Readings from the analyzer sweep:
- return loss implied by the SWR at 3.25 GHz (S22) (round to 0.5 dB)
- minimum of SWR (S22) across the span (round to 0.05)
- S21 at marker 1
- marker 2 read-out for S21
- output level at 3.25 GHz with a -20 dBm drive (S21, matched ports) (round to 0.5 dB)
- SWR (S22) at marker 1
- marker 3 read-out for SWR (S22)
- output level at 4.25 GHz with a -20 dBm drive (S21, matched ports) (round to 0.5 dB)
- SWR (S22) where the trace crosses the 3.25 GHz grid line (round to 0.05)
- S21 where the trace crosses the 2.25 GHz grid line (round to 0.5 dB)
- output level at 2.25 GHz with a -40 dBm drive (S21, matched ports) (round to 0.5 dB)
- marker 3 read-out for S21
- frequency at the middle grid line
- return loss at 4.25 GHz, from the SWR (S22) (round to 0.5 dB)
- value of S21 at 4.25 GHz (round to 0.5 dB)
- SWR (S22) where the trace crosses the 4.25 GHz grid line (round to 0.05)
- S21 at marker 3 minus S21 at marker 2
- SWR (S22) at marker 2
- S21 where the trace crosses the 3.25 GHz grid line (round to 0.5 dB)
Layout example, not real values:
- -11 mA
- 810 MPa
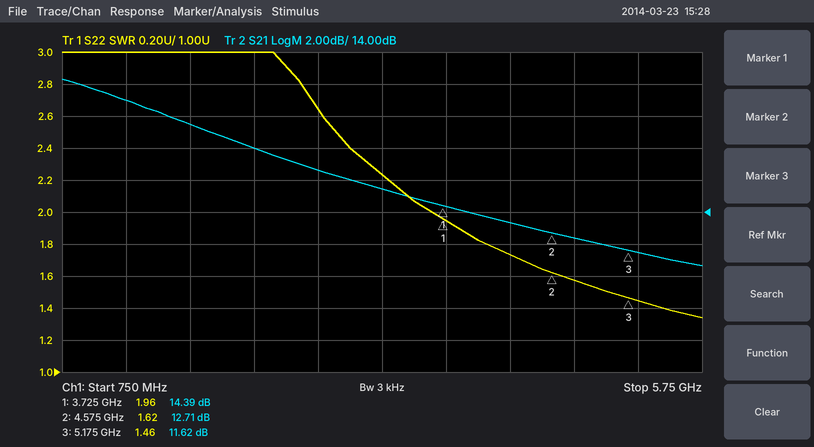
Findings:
- 8.5 dB
- 1.35
- 14.39 dB
- 12.71 dB
- -4.5 dBm
- 1.96
- 1.46
- -6.5 dBm
- 2.25
- 18.0 dB
- -22.0 dBm
- 11.62 dB
- 3.25 GHz
- 11.5 dB
- 13.5 dB
- 1.75
- -1.09 dB
- 1.62
- 15.5 dB
